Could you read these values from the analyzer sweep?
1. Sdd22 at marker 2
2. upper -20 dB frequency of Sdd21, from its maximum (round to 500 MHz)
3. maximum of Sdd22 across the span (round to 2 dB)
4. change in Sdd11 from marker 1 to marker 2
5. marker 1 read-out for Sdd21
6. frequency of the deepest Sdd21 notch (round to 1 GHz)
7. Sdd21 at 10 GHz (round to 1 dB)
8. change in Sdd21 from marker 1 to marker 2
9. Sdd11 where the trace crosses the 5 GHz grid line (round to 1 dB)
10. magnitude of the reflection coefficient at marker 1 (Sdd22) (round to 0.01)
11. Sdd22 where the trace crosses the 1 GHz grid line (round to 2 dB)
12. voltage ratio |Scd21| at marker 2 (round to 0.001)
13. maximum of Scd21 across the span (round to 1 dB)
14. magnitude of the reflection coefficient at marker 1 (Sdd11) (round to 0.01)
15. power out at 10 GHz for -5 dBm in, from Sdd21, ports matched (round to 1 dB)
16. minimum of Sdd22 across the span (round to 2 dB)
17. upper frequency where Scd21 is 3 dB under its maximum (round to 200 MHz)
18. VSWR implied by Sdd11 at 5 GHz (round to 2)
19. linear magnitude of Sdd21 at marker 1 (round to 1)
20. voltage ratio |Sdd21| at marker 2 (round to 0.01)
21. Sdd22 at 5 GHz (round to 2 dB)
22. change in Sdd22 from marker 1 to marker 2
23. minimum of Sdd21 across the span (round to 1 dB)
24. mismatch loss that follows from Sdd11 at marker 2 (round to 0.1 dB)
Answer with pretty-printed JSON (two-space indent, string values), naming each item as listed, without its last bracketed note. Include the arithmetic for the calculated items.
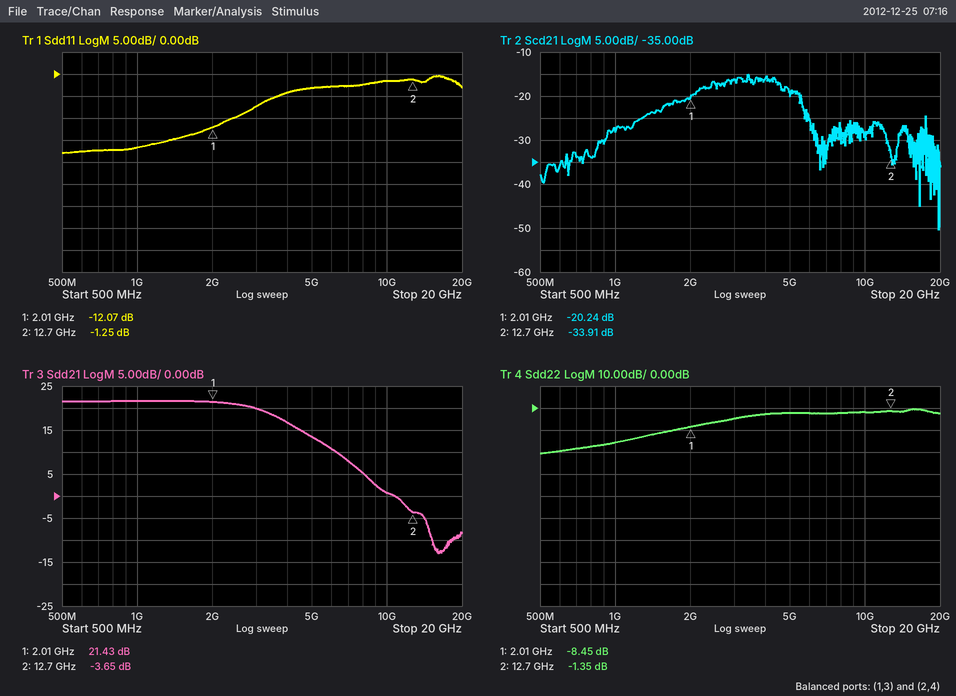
{
  "Sdd22 at marker 2": "-1.35 dB",
  "upper -20 dB frequency of Sdd21, from its maximum": "9.5 GHz",
  "maximum of Sdd22 across the span": "0 dB",
  "change in Sdd11 from marker 1 to marker 2": "-1.25 − (-12.07) = 10.82 dB",
  "marker 1 read-out for Sdd21": "21.43 dB",
  "frequency of the deepest Sdd21 notch": "16 GHz",
  "Sdd21 at 10 GHz": "1 dB",
  "change in Sdd21 from marker 1 to marker 2": "-3.65 − (21.43) = -25.08 dB",
  "Sdd11 where the trace crosses the 5 GHz grid line": "-3 dB",
  "magnitude of the reflection coefficient at marker 1 (Sdd22)": "10^(-8.45/20) ≈ 0.38",
  "Sdd22 where the trace crosses the 1 GHz grid line": "-16 dB",
  "voltage ratio |Scd21| at marker 2": "10^(-33.91/20) ≈ 0.020",
  "maximum of Scd21 across the span": "-15 dB",
  "magnitude of the reflection coefficient at marker 1 (Sdd11)": "10^(-12.07/20) ≈ 0.25",
  "power out at 10 GHz for -5 dBm in, from Sdd21, ports matched": "-5 dBm + (1 dB) = -4 dBm",
  "minimum of Sdd22 across the span": "-20 dB",
  "upper frequency where Scd21 is 3 dB under its maximum": "4.6 GHz",
  "VSWR implied by Sdd11 at 5 GHz": "|Γ| = 10^(-3/20) = 0.7079; VSWR = (1 + 0.7079)/(1 − 0.7079) ≈ 6",
  "linear magnitude of Sdd21 at marker 1": "10^(21.43/20) ≈ 12",
  "voltage ratio |Sdd21| at marker 2": "10^(-3.65/20) ≈ 0.66",
  "Sdd22 at 5 GHz": "-2 dB",
  "change in Sdd22 from marker 1 to marker 2": "-1.35 − (-8.45) = 7.10 dB",
  "minimum of Sdd21 across the span": "-13 dB",
  "mismatch loss that follows from Sdd11 at marker 2": "−10 log10(1 − 10^(-1.25/10)) ≈ 6.0 dB"
}
